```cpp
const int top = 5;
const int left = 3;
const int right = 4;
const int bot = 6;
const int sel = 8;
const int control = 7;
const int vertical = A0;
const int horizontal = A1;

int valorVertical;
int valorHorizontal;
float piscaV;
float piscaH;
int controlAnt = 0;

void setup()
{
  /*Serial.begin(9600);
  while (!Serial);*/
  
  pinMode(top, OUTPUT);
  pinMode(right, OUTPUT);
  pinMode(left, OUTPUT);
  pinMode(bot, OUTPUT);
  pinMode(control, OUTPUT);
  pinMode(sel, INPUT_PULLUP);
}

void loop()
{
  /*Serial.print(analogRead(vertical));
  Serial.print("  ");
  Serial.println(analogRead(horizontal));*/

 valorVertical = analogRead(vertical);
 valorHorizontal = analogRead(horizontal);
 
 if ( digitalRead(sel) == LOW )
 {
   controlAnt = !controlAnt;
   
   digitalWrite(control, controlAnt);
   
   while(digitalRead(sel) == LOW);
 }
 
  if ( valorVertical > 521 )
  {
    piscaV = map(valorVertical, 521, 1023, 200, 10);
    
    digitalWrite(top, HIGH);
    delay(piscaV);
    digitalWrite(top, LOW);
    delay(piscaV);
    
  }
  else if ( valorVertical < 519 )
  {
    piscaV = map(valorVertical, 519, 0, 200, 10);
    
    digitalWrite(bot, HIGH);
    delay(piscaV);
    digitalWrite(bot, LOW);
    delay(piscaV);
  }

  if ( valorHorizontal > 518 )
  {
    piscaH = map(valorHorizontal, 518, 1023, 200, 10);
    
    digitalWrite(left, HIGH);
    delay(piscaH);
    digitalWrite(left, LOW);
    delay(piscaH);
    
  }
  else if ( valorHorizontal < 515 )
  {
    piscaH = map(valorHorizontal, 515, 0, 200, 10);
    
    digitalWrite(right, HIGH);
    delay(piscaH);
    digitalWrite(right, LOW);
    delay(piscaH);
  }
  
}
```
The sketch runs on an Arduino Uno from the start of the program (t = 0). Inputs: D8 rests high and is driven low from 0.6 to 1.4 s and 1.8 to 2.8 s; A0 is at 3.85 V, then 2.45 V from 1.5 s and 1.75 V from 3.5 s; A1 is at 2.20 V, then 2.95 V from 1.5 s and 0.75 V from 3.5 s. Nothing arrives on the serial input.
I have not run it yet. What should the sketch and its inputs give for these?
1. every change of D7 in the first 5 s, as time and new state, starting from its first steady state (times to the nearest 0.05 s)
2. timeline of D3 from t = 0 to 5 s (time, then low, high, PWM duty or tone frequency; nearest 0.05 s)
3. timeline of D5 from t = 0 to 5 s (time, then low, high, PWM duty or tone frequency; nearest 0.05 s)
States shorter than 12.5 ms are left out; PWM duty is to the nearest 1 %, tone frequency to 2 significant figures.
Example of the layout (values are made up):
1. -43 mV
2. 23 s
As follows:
1. 0 s low; 1.1 s high; 1.95 s low
2. 0 s low; 3.2 s high; 3.35 s low
3. 0 s high; 0.1 s low; 0.55 s high; 0.65 s low; 1.4 s high; 1.5 s low
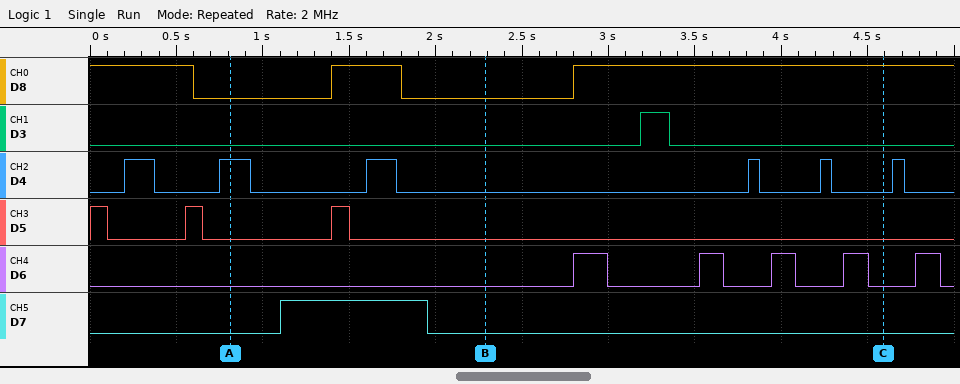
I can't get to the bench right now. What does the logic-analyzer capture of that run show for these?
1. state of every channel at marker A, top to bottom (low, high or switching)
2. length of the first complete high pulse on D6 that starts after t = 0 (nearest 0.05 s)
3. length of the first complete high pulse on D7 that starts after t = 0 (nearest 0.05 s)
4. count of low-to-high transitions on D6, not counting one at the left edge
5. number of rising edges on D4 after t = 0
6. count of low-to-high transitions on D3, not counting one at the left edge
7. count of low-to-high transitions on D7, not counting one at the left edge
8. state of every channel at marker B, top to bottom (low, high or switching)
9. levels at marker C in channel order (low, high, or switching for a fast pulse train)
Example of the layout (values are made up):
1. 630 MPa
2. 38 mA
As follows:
1. D8 low, D3 low, D4 high, D5 low, D6 low, D7 low
2. 0.20 s
3. 0.85 s
4. 5
5. 6
6. 1
7. 1
8. D8 low, D3 low, D4 low, D5 low, D6 low, D7 low
9. D8 high, D3 low, D4 low, D5 low, D6 low, D7 low
